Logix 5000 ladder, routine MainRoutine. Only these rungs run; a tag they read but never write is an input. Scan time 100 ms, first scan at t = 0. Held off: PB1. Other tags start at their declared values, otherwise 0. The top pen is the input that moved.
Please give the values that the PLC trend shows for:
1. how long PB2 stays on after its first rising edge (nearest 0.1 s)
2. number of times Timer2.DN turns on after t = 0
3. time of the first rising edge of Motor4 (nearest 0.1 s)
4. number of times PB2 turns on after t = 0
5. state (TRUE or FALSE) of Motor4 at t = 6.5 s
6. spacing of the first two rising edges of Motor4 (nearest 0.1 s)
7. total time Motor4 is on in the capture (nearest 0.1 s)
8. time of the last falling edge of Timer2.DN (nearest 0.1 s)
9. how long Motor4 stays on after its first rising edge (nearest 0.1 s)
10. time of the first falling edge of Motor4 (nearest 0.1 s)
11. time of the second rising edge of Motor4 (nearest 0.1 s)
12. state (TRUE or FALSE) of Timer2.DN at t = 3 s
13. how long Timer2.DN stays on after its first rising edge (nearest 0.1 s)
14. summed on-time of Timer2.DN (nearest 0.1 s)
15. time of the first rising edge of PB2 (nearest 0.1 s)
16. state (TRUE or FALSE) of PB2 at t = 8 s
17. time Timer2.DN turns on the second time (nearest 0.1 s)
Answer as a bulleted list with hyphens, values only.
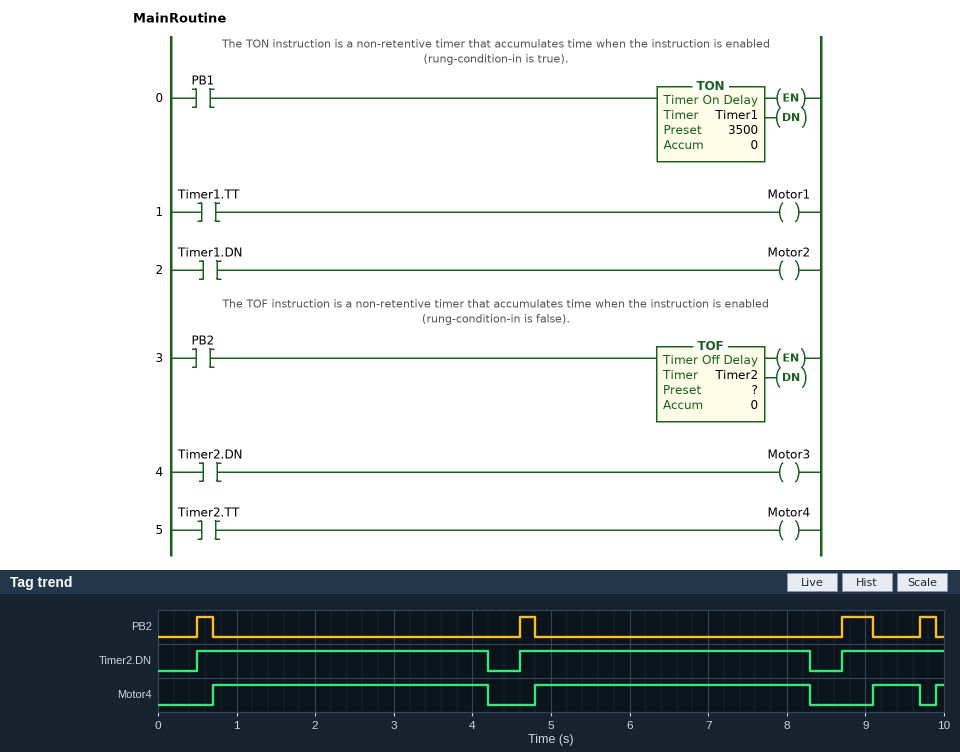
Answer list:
- 0.2 s
- 3
- 0.7 s
- 4
- TRUE
- 4.1 s
- 7.7 s
- 8.3 s
- 3.5 s
- 4.2 s
- 4.8 s
- TRUE
- 3.7 s
- 8.7 s
- 0.5 s
- FALSE
- 4.6 s
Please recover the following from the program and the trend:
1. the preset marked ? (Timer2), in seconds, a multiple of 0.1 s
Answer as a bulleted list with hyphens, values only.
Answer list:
- 3.5 s
